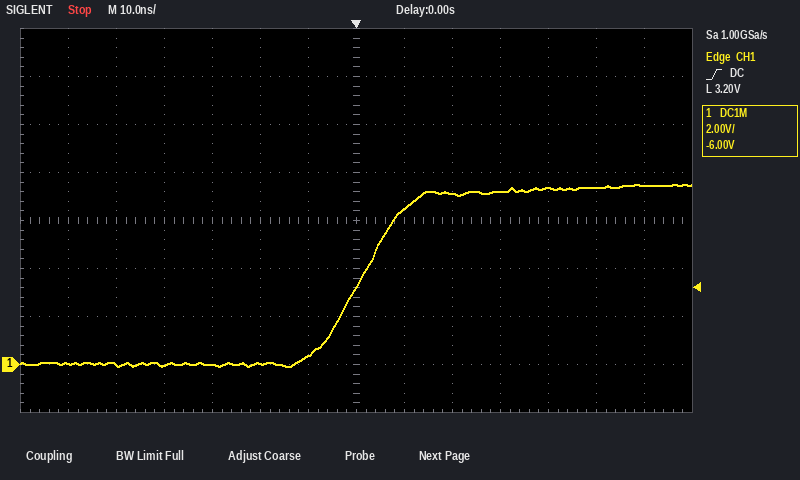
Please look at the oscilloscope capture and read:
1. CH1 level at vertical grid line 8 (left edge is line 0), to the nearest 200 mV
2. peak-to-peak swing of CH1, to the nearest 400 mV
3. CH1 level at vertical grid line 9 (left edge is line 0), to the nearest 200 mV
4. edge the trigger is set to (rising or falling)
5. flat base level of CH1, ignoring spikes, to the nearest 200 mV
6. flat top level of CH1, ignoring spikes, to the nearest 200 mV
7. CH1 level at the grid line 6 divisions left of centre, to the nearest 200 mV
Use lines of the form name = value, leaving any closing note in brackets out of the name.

CH1 level at vertical grid line 8 (left edge is line 0), to the nearest 200 mV = 6.4 V
peak-to-peak swing of CH1, to the nearest 400 mV = 7.6 V
CH1 level at vertical grid line 9 (left edge is line 0), to the nearest 200 mV = 7.2 V
edge the trigger is set to = rising
flat base level of CH1, ignoring spikes, to the nearest 200 mV = 0.0 V
flat top level of CH1, ignoring spikes, to the nearest 200 mV = 7.4 V
CH1 level at the grid line 6 divisions left of centre, to the nearest 200 mV = 0.0 V
